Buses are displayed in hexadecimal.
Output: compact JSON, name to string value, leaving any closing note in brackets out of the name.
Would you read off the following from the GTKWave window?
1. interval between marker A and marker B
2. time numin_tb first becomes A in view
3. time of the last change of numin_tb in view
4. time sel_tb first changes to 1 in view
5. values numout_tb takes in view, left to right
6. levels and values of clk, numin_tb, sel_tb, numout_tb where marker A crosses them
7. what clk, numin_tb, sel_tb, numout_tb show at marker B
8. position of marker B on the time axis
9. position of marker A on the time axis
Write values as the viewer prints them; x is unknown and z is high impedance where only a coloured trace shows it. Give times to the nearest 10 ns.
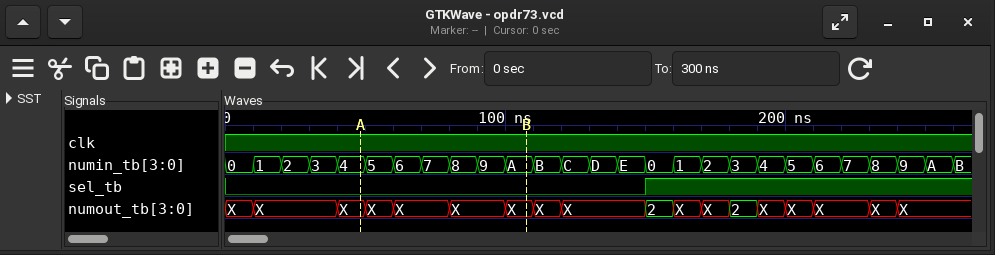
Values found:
{"interval between marker A and marker B": "60 ns", "time numin_tb first becomes A in view": "100 ns", "time of the last change of numin_tb in view": "260 ns", "time sel_tb first changes to 1 in view": "150 ns", "values numout_tb takes in view, left to right": "X, X, X, X, X, X, X, X, X, 2, X, X, 2, X, X, X, X, X", "levels and values of clk, numin_tb, sel_tb, numout_tb where marker A crosses them": "clk=1, numin_tb=4, sel_tb=0, numout_tb=X", "what clk, numin_tb, sel_tb, numout_tb show at marker B": "clk=1, numin_tb=A, sel_tb=0, numout_tb=X", "position of marker B on the time axis": "110 ns", "position of marker A on the time axis": "50 ns"}
